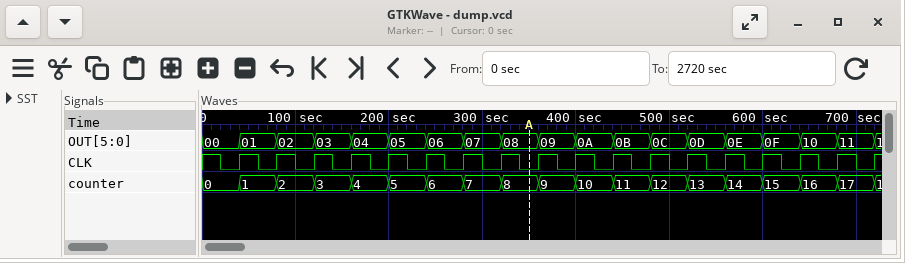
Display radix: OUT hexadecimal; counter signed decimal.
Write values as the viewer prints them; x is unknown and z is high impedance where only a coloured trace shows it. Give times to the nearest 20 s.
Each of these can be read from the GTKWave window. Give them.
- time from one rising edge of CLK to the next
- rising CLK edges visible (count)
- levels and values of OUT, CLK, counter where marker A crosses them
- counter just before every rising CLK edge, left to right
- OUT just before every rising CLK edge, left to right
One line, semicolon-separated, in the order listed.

40 s; 18; OUT=08, CLK=0, counter=8; 0, 1, 2, 3, 4, 5, 6, 7, 8, 9, 10, 11, 12, 13, 14, 15, 16, 17; 00, 01, 02, 03, 04, 05, 06, 07, 08, 09, 0A, 0B, 0C, 0D, 0E, 0F, 10, 11
